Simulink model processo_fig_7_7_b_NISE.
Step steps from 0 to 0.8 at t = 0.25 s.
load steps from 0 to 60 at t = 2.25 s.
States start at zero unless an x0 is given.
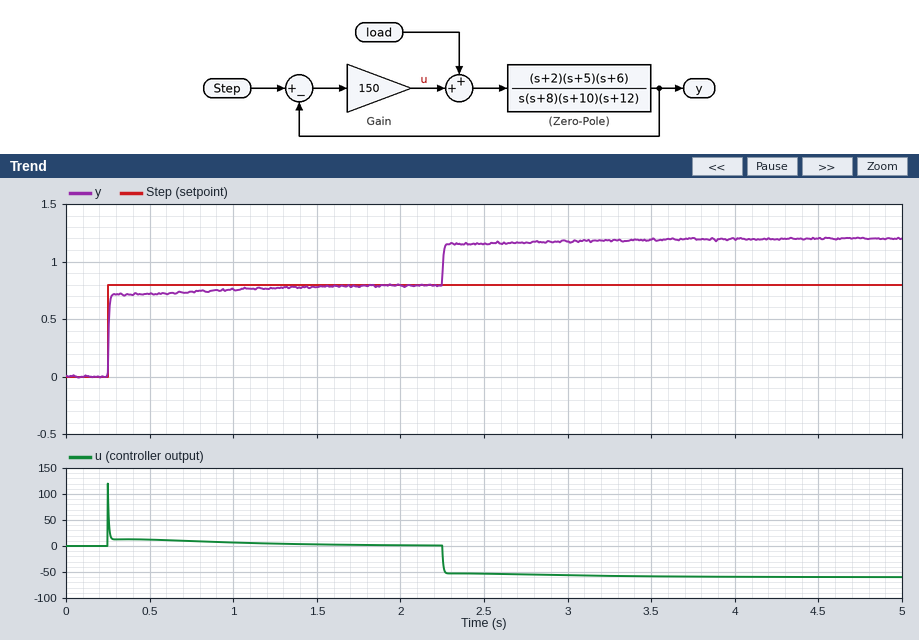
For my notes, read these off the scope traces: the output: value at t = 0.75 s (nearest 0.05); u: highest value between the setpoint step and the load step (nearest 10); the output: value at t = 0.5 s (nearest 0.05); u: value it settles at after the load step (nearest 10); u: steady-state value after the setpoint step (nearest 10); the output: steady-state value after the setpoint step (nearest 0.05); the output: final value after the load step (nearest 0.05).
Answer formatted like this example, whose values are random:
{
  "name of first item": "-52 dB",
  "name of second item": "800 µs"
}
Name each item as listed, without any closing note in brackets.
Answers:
{
  "the output: value at t = 0.75 s": "0.75",
  "u: highest value between the setpoint step and the load step": "120",
  "the output: value at t = 0.5 s": "0.70",
  "u: value it settles at after the load step": "-60",
  "u: steady-state value after the setpoint step": "0",
  "the output: steady-state value after the setpoint step": "0.80",
  "the output: final value after the load step": "1.20"
}
